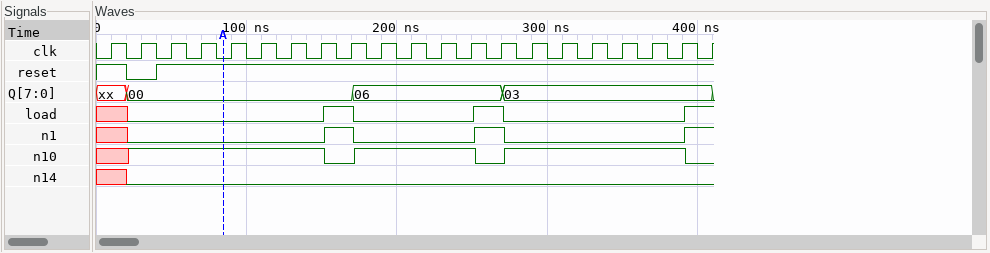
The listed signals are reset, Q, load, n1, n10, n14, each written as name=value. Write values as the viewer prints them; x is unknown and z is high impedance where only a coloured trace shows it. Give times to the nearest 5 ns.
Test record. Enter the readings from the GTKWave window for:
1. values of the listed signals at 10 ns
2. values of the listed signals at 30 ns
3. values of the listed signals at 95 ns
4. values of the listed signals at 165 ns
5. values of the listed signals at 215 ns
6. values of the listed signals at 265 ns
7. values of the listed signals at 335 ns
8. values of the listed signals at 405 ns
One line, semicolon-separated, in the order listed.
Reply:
reset=1, Q=xx, load=x, n1=x, n10=x, n14=x; reset=0, Q=00, load=0, n1=0, n10=1, n14=0; reset=1, Q=00, load=0, n1=0, n10=1, n14=0; reset=1, Q=00, load=1, n1=1, n10=0, n14=0; reset=1, Q=06, load=0, n1=0, n10=1, n14=0; reset=1, Q=06, load=1, n1=1, n10=0, n14=0; reset=1, Q=03, load=0, n1=0, n10=1, n14=0; reset=1, Q=03, load=1, n1=1, n10=0, n14=0
